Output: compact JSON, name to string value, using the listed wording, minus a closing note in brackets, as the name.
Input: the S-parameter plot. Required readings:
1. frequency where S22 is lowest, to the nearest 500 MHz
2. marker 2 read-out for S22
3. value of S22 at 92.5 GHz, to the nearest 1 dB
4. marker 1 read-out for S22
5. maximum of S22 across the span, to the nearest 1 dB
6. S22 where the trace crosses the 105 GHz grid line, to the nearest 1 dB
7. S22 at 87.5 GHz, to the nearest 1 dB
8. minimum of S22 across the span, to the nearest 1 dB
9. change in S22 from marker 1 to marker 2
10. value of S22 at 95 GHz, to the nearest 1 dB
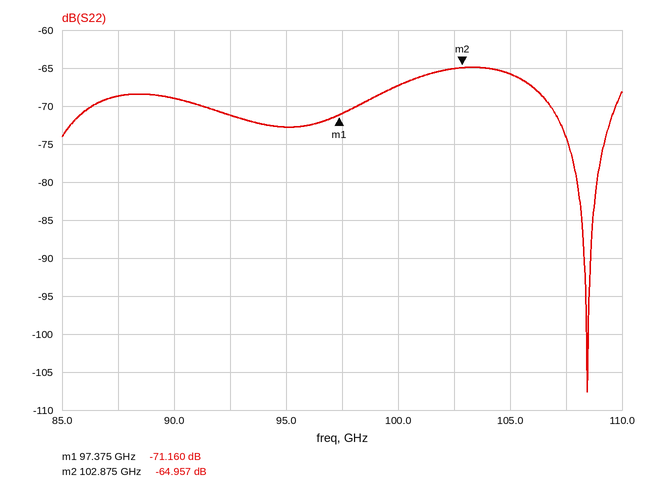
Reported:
{"frequency where S22 is lowest, to the nearest 500 MHz": "108.5 GHz", "marker 2 read-out for S22": "-64.957 dB", "value of S22 at 92.5 GHz, to the nearest 1 dB": "-71 dB", "marker 1 read-out for S22": "-71.160 dB", "maximum of S22 across the span, to the nearest 1 dB": "-65 dB", "S22 where the trace crosses the 105 GHz grid line, to the nearest 1 dB": "-66 dB", "S22 at 87.5 GHz, to the nearest 1 dB": "-69 dB", "minimum of S22 across the span, to the nearest 1 dB": "-108 dB", "change in S22 from marker 1 to marker 2": "6.203 dB", "value of S22 at 95 GHz, to the nearest 1 dB": "-73 dB"}
